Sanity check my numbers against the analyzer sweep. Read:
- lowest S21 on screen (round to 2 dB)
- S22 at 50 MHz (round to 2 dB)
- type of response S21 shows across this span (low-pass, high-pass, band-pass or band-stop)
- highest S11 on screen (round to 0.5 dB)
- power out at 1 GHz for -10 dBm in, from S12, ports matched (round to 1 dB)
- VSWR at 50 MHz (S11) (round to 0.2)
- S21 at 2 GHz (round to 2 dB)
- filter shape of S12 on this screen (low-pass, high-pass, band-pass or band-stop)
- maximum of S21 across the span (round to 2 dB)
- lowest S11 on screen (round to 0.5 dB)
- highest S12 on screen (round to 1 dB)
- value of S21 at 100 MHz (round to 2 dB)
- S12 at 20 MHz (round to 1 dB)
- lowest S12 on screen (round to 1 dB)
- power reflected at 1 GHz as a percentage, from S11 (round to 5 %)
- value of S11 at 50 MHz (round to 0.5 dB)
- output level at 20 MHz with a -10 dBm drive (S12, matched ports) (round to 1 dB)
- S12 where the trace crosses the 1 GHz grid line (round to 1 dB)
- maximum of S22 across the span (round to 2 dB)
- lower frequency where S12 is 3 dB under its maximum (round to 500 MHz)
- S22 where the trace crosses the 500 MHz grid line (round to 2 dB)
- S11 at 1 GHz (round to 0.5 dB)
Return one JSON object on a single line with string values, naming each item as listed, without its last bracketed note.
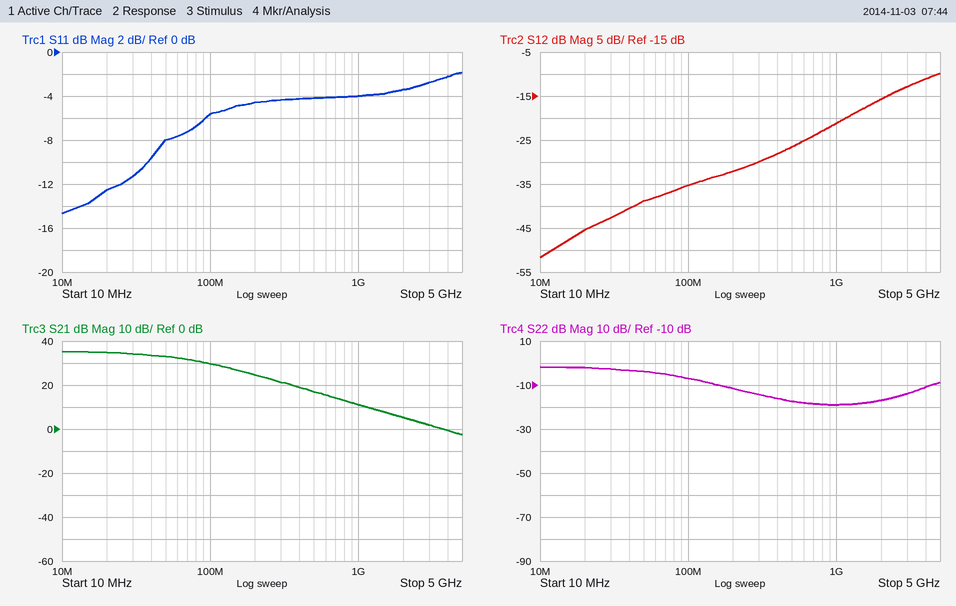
{"lowest S21 on screen": "-2 dB", "S22 at 50 MHz": "-4 dB", "type of response S21 shows across this span": "low-pass", "highest S11 on screen": "-2.0 dB", "power out at 1 GHz for -10 dBm in, from S12, ports matched": "-31 dBm", "VSWR at 50 MHz (S11)": "2.4", "S21 at 2 GHz": "6 dB", "filter shape of S12 on this screen": "high-pass", "maximum of S21 across the span": "36 dB", "lowest S11 on screen": "-14.5 dB", "highest S12 on screen": "-10 dB", "value of S21 at 100 MHz": "30 dB", "S12 at 20 MHz": "-45 dB", "lowest S12 on screen": "-52 dB", "power reflected at 1 GHz as a percentage, from S11": "40 %", "value of S11 at 50 MHz": "-8.0 dB", "output level at 20 MHz with a -10 dBm drive (S12, matched ports)": "-55 dBm", "S12 where the trace crosses the 1 GHz grid line": "-21 dB", "maximum of S22 across the span": "-2 dB", "lower frequency where S12 is 3 dB under its maximum": "3.0 GHz", "S22 where the trace crosses the 500 MHz grid line": "-18 dB", "S11 at 1 GHz": "-4.0 dB"}
